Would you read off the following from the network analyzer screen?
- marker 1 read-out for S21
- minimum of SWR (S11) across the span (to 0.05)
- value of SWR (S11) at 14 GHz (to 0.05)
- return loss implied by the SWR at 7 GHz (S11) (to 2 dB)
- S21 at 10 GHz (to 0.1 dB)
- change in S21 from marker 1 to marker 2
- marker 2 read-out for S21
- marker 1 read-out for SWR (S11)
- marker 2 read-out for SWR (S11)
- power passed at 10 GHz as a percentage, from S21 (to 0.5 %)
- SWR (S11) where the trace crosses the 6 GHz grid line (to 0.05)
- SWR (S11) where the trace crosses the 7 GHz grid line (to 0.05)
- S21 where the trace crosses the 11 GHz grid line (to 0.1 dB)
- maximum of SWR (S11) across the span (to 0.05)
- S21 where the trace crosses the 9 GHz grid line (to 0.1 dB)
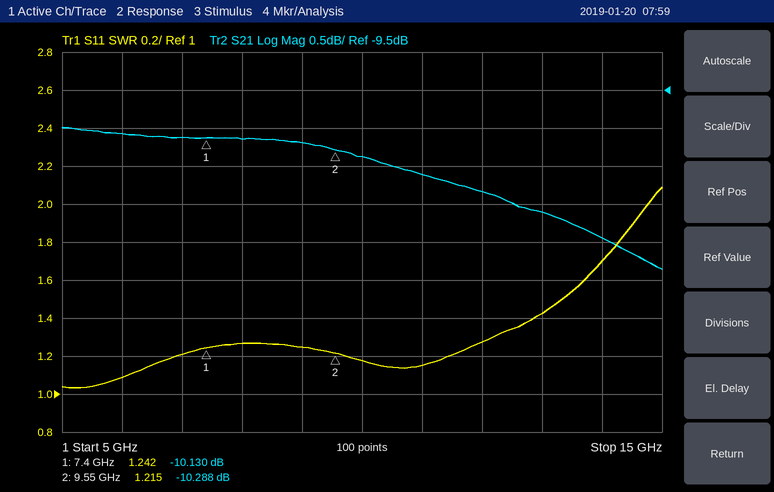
-10.130 dB
1.05
1.70
20 dB
-10.4 dB
-0.158 dB
-10.288 dB
1.242
1.215
9.0 %
1.10
1.20
-10.6 dB
2.10
-10.2 dB
